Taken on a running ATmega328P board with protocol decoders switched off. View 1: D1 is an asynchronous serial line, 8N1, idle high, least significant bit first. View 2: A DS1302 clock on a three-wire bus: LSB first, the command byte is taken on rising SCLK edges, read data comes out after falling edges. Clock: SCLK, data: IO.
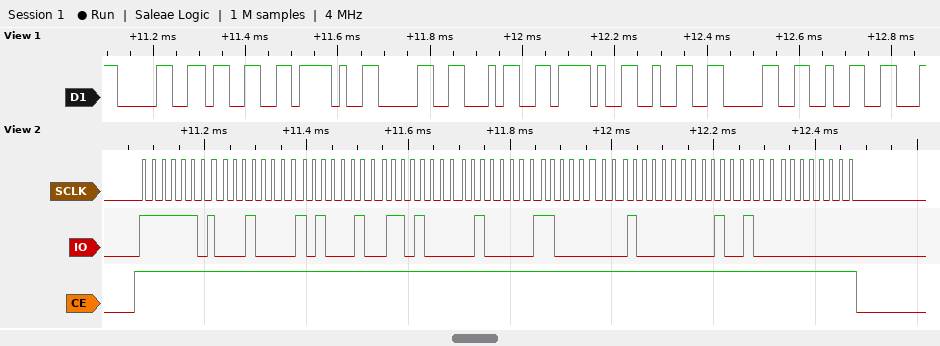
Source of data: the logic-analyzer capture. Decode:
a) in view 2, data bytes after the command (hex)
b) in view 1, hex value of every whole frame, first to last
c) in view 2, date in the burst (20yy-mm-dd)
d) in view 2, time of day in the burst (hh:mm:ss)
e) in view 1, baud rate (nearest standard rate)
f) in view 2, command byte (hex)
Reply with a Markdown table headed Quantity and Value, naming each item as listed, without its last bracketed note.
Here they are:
| Quantity | Value |
|---|---|
| in view 2, data bytes after the command | 08 45 16 04 03 02 24 00 |
| in view 1, hex value of every whole frame, first to last | 30 33 2F 30 34 2F 32 30 32 |
| in view 2, date in the burst | 2024-03-04 |
| in view 2, time of day in the burst | 16:45:08 |
| in view 1, baud rate | 57600 baud |
| in view 2, command byte | 0xBF |
